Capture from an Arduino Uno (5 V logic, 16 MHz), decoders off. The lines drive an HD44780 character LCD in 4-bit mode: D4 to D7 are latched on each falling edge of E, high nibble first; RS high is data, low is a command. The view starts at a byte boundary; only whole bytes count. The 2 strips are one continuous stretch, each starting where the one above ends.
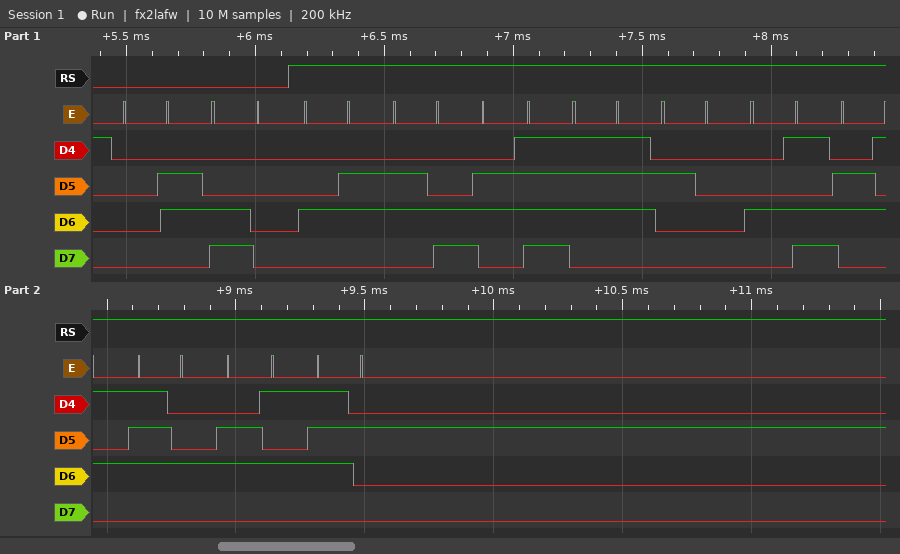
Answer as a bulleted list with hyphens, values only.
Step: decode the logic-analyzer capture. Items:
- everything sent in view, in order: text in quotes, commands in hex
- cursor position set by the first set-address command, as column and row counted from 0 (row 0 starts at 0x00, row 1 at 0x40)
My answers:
- 0x06 0xC0 "Flow Meter"
- column 0, row 1
